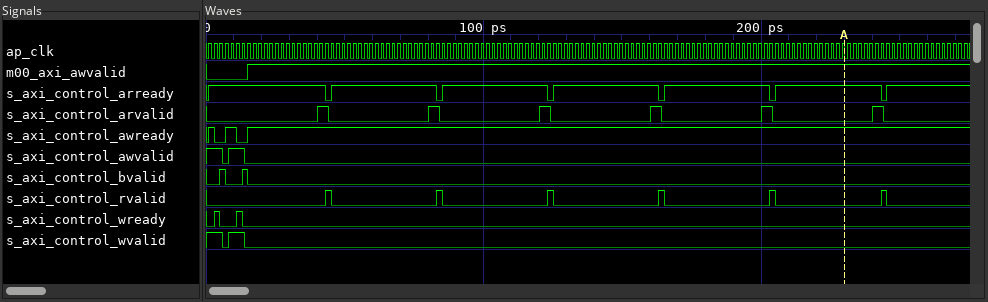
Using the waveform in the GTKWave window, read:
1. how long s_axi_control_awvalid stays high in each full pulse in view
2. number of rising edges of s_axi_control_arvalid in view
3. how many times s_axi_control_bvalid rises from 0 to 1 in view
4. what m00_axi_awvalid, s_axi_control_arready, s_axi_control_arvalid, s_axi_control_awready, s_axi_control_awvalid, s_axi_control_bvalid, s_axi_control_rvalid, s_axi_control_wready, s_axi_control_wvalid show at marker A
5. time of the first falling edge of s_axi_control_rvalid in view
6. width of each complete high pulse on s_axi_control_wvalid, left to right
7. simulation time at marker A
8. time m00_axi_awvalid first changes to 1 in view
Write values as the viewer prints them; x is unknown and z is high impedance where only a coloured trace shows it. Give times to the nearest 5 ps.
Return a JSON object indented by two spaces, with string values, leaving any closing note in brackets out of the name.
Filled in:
{
  "how long s_axi_control_awvalid stays high in each full pulse in view": "5 ps",
  "number of rising edges of s_axi_control_arvalid in view": "6",
  "how many times s_axi_control_bvalid rises from 0 to 1 in view": "2",
  "what m00_axi_awvalid, s_axi_control_arready, s_axi_control_arvalid, s_axi_control_awready, s_axi_control_awvalid, s_axi_control_bvalid, s_axi_control_rvalid, s_axi_control_wready, s_axi_control_wvalid show at marker A": "m00_axi_awvalid=1, s_axi_control_arready=1, s_axi_control_arvalid=0, s_axi_control_awready=1, s_axi_control_awvalid=0, s_axi_control_bvalid=0, s_axi_control_rvalid=0, s_axi_control_wready=0, s_axi_control_wvalid=0",
  "time of the first falling edge of s_axi_control_rvalid in view": "45 ps",
  "width of each complete high pulse on s_axi_control_wvalid, left to right": "5 ps",
  "simulation time at marker A": "230 ps",
  "time m00_axi_awvalid first changes to 1 in view": "15 ps"
}
